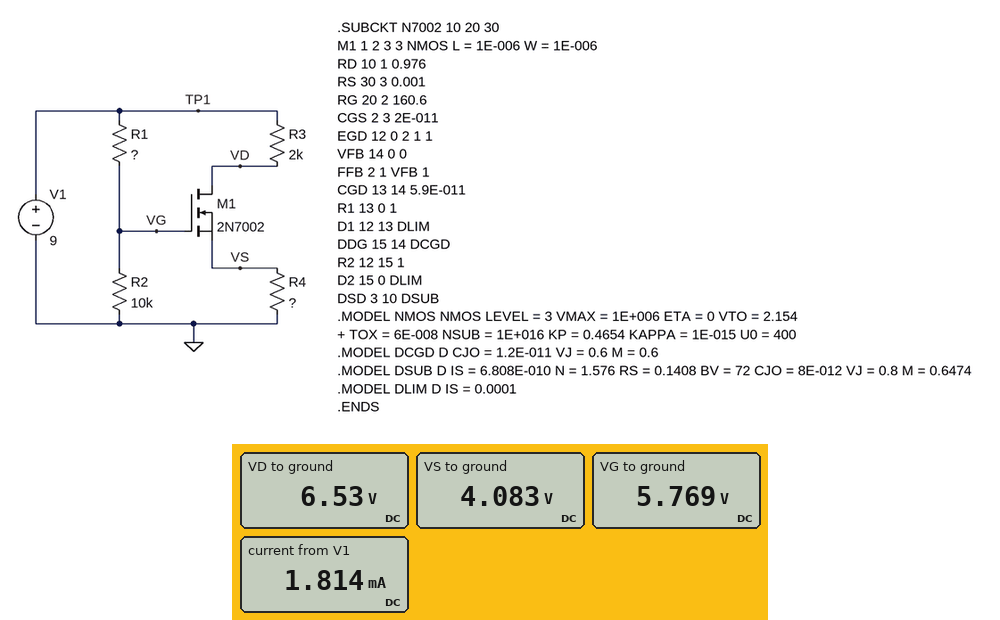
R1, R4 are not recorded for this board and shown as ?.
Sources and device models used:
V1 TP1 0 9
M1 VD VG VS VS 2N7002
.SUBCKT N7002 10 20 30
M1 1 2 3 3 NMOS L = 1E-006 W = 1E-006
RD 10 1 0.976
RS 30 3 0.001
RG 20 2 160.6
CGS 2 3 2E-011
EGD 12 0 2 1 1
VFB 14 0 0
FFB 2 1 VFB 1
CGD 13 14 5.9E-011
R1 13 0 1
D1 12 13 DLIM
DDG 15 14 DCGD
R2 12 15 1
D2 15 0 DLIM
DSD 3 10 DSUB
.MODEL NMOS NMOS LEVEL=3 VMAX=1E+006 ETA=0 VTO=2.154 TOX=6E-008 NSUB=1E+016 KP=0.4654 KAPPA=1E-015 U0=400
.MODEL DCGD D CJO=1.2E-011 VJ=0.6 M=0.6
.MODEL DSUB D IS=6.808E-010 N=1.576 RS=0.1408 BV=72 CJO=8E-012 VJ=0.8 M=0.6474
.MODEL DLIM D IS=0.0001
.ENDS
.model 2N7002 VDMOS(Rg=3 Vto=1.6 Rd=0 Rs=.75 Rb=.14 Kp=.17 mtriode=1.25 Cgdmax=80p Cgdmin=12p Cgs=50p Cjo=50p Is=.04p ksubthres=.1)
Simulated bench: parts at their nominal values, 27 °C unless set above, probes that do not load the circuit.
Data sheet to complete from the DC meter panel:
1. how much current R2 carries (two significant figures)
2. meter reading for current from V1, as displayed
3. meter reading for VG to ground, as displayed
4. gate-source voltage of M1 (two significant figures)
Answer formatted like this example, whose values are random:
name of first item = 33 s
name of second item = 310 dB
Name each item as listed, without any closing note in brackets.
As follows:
how much current R2 carries = 580 µA
meter reading for current from V1, as displayed = 1.814 mA
meter reading for VG to ground, as displayed = 5.769 V
gate-source voltage of M1 = 1.7 V
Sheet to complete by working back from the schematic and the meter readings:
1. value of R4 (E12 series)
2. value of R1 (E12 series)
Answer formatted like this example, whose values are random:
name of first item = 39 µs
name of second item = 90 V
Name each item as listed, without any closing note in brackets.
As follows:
value of R4 = 3.3 kΩ
value of R1 = 5.6 kΩ
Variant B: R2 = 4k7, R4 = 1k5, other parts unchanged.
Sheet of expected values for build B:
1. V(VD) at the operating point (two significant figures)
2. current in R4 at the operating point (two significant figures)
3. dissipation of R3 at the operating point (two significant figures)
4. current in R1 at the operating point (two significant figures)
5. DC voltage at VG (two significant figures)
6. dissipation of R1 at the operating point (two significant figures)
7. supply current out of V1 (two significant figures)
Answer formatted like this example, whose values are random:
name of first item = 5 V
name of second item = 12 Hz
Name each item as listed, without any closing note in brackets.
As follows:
V(VD) at the operating point = 5.8 V
current in R4 at the operating point = 1.6 mA
dissipation of R3 at the operating point = 5.1 mW
current in R1 at the operating point = 870 µA
DC voltage at VG = 4.1 V
dissipation of R1 at the operating point = 4.3 mW
supply current out of V1 = 2.5 mA
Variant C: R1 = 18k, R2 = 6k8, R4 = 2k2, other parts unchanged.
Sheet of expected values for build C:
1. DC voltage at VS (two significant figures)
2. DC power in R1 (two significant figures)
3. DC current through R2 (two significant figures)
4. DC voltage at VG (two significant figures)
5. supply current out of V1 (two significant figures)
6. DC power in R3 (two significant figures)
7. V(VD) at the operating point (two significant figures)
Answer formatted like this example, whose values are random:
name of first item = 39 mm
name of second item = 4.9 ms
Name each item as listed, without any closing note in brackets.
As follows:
DC voltage at VS = 870 mV
DC power in R1 = 2.4 mW
DC current through R2 = 360 µA
DC voltage at VG = 2.5 V
supply current out of V1 = 760 µA
DC power in R3 = 310 µW
V(VD) at the operating point = 8.2 V
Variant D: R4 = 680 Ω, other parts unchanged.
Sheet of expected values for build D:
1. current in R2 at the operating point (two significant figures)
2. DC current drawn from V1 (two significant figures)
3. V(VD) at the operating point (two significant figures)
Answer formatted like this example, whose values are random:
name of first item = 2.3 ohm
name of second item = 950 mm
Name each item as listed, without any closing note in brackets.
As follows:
current in R2 at the operating point = 580 µA
DC current drawn from V1 = 3.9 mA
V(VD) at the operating point = 2.3 V
